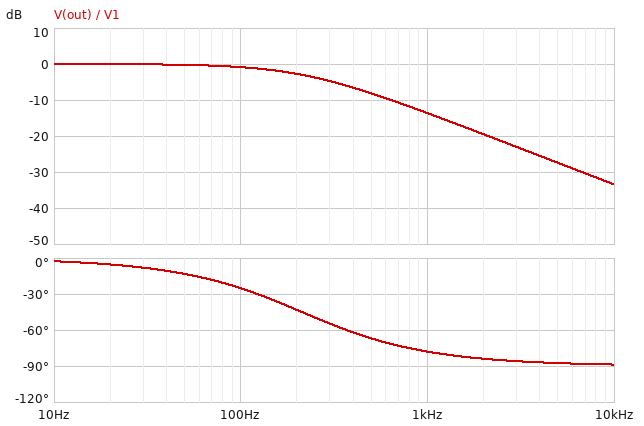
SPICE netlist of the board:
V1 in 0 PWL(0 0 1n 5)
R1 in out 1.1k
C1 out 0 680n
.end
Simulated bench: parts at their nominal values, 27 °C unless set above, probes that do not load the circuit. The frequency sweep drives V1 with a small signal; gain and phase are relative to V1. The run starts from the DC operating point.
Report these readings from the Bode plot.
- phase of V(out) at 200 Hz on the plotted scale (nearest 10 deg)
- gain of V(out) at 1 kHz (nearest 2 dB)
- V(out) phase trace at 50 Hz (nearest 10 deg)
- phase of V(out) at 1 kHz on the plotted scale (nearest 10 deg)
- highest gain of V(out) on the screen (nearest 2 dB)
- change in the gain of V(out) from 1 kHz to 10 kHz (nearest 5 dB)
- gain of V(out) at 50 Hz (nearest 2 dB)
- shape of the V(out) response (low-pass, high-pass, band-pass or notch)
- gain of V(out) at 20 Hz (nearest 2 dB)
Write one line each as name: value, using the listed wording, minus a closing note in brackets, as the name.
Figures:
phase of V(out) at 200 Hz on the plotted scale: -40 deg
gain of V(out) at 1 kHz: -14 dB
V(out) phase trace at 50 Hz: -10 deg
phase of V(out) at 1 kHz on the plotted scale: -80 deg
highest gain of V(out) on the screen: 0 dB
change in the gain of V(out) from 1 kHz to 10 kHz: -20 dB
gain of V(out) at 50 Hz: 0 dB
shape of the V(out) response: low-pass
gain of V(out) at 20 Hz: 0 dB
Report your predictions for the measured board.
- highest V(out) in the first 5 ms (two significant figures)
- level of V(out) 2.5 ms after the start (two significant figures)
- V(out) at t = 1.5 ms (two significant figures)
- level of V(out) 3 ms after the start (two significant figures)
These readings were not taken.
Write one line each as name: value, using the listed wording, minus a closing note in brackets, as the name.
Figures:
highest V(out) in the first 5 ms: 5.0 V
level of V(out) 2.5 ms after the start: 4.8 V
V(out) at t = 1.5 ms: 4.3 V
level of V(out) 3 ms after the start: 4.9 V
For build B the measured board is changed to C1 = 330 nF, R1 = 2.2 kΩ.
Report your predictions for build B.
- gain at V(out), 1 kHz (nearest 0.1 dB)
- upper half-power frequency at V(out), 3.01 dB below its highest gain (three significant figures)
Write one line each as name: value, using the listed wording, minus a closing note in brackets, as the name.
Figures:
gain at V(out), 1 kHz: -13.4 dB
upper half-power frequency at V(out), 3.01 dB below its highest gain: 219 Hz
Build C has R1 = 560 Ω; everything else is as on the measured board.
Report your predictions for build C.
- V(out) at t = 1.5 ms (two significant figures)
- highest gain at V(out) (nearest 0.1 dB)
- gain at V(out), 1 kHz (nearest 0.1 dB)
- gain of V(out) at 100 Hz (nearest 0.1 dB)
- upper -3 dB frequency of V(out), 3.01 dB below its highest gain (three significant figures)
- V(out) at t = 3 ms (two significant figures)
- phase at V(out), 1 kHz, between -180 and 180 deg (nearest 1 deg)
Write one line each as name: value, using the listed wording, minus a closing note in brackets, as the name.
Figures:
V(out) at t = 1.5 ms: 4.9 V
highest gain at V(out): 0 dB
gain at V(out), 1 kHz: -8.3 dB
gain of V(out) at 100 Hz: -0.2 dB
upper -3 dB frequency of V(out), 3.01 dB below its highest gain: 418 Hz
V(out) at t = 3 ms: 5.0 V
phase at V(out), 1 kHz, between -180 and 180 deg: -67 deg
